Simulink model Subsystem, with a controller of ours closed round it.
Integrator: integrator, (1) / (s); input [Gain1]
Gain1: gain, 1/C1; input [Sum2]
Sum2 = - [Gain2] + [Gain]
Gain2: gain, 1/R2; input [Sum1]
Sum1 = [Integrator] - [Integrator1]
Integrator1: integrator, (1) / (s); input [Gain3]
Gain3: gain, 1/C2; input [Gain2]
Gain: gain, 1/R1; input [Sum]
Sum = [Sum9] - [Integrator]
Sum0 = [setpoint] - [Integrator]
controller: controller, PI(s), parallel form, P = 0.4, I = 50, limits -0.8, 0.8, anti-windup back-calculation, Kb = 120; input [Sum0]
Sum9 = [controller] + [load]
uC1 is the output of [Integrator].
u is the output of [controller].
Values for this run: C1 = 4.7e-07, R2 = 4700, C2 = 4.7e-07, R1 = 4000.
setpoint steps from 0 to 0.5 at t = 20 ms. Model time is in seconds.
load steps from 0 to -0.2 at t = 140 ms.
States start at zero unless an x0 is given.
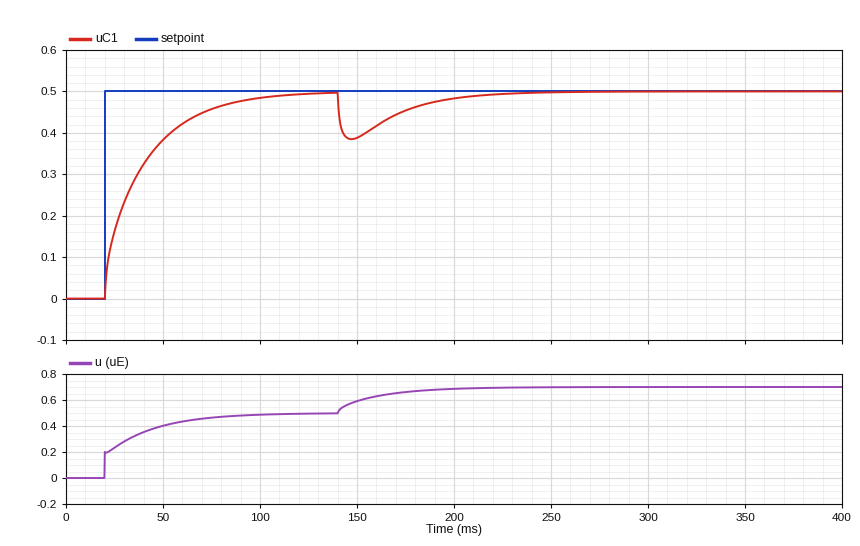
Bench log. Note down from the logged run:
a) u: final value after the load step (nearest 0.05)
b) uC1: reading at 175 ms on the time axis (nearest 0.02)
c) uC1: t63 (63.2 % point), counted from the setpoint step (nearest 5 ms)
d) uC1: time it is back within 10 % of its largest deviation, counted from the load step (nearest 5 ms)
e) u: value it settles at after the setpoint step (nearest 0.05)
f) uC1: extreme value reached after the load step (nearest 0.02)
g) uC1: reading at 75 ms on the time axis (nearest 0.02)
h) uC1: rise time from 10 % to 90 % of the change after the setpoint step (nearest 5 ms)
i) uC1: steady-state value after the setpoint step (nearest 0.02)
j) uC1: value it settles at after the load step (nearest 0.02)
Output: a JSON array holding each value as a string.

["0.70", "0.46", "20 ms", "70 ms", "0.50", "0.38", "0.46", "50 ms", "0.50", "0.50"]
